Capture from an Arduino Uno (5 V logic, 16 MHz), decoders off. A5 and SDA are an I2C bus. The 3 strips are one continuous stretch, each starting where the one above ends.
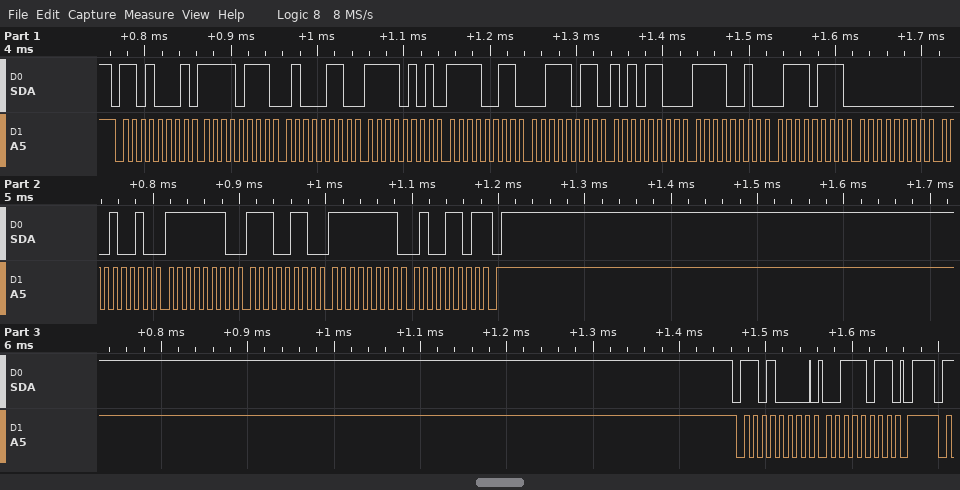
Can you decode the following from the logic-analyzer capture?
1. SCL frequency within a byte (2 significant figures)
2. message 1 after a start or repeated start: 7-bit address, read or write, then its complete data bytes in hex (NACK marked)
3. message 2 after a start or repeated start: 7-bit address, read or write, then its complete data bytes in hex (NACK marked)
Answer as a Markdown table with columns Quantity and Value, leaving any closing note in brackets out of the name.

| Quantity | Value |
|---|---|
| SCL frequency within a byte | 100 kHz |
| message 1 after a start or repeated start: 7-bit address, read or write, then its complete data bytes in hex | 0x68 read: F7 46 F5 F3 3B AC F2 77 00 12 FE E6 FF 4D NACK |
| message 2 after a start or repeated start: 7-bit address, read or write, then its complete data bytes in hex | 0x68 write: 3B |
